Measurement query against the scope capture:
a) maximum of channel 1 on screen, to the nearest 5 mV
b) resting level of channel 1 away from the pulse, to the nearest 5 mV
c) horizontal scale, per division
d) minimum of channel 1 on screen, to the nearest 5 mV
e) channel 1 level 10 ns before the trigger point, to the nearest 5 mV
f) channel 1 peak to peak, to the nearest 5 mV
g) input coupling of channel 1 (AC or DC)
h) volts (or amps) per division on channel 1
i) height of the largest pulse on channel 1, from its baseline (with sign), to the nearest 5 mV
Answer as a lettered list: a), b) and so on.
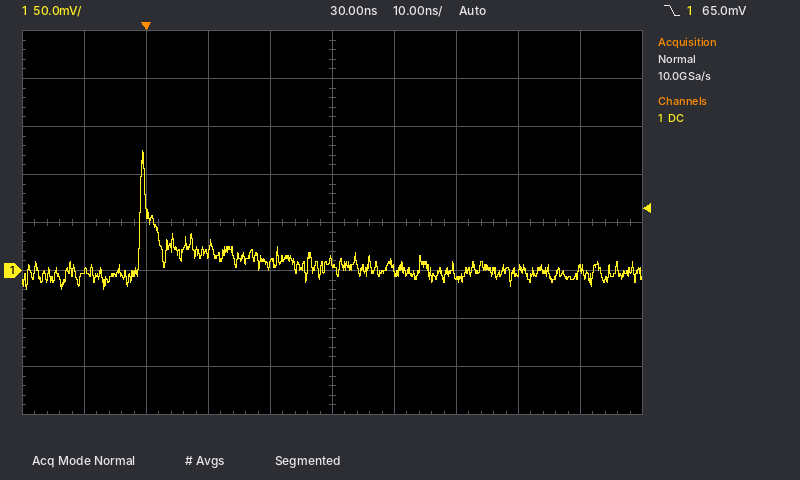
a) 125 mV
b) 0 mV
c) 10 ns
d) -20 mV
e) 0 mV
f) 145 mV
g) DC
h) 50 mV
i) +125 mV
